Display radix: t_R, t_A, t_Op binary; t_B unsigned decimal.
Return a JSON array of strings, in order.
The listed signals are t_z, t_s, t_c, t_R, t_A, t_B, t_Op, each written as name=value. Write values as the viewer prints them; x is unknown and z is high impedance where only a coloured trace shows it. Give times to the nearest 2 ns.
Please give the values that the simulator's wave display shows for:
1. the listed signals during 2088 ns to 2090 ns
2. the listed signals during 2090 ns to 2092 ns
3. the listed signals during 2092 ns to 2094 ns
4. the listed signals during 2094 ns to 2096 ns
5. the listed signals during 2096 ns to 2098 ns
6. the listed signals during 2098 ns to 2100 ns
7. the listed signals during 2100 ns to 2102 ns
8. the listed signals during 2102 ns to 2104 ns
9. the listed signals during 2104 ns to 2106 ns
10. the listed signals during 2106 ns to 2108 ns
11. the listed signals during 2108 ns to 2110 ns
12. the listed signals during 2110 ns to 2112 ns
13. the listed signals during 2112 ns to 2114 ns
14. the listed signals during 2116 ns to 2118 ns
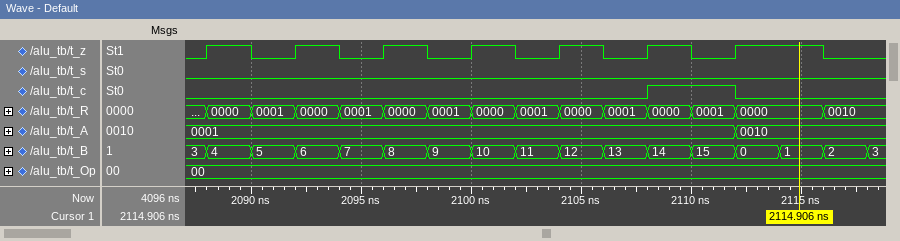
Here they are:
["t_z=1, t_s=0, t_c=0, t_R=0000, t_A=0001, t_B=4, t_Op=00", "t_z=0, t_s=0, t_c=0, t_R=0001, t_A=0001, t_B=5, t_Op=00", "t_z=1, t_s=0, t_c=0, t_R=0000, t_A=0001, t_B=6, t_Op=00", "t_z=0, t_s=0, t_c=0, t_R=0001, t_A=0001, t_B=7, t_Op=00", "t_z=1, t_s=0, t_c=0, t_R=0000, t_A=0001, t_B=8, t_Op=00", "t_z=0, t_s=0, t_c=0, t_R=0001, t_A=0001, t_B=9, t_Op=00", "t_z=1, t_s=0, t_c=0, t_R=0000, t_A=0001, t_B=10, t_Op=00", "t_z=0, t_s=0, t_c=0, t_R=0001, t_A=0001, t_B=11, t_Op=00", "t_z=1, t_s=0, t_c=0, t_R=0000, t_A=0001, t_B=12, t_Op=00", "t_z=0, t_s=0, t_c=0, t_R=0001, t_A=0001, t_B=13, t_Op=00", "t_z=1, t_s=0, t_c=1, t_R=0000, t_A=0001, t_B=14, t_Op=00", "t_z=0, t_s=0, t_c=1, t_R=0001, t_A=0001, t_B=15, t_Op=00", "t_z=1, t_s=0, t_c=0, t_R=0000, t_A=0010, t_B=0, t_Op=00", "t_z=0, t_s=0, t_c=0, t_R=0010, t_A=0010, t_B=2, t_Op=00"]
